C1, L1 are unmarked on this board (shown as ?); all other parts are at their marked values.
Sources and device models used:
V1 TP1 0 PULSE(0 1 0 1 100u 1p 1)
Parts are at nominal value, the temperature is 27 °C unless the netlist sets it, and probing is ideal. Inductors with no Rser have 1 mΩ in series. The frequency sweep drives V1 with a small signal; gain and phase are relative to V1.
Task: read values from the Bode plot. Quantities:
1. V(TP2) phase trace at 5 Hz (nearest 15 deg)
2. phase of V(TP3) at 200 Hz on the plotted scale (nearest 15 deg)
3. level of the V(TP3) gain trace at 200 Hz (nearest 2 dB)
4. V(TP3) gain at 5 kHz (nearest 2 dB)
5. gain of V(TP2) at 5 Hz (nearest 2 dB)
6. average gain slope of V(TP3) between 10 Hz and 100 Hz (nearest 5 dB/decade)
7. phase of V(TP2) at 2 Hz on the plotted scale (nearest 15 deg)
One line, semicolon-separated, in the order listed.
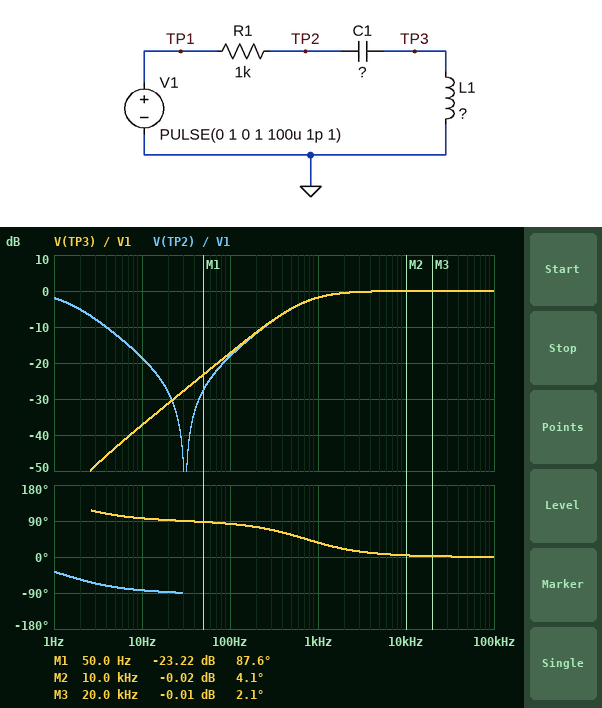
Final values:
-75 deg; 75 deg; -12 dB; 0 dB; -12 dB; 20 dB/decade; -60 deg
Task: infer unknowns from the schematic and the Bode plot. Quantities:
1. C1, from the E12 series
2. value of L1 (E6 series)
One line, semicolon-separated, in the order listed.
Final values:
120 µF; 220 mH
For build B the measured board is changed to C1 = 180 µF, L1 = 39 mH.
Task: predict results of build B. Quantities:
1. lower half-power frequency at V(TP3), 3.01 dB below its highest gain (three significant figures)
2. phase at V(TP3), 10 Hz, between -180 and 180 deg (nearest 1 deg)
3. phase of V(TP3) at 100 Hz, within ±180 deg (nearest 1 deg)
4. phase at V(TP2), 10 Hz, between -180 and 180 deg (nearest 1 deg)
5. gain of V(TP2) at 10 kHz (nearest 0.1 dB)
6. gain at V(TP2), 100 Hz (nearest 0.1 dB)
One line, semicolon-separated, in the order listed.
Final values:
4.08 kHz; 95 deg; 89 deg; -85 deg; -0.7 dB; -36.1 dB
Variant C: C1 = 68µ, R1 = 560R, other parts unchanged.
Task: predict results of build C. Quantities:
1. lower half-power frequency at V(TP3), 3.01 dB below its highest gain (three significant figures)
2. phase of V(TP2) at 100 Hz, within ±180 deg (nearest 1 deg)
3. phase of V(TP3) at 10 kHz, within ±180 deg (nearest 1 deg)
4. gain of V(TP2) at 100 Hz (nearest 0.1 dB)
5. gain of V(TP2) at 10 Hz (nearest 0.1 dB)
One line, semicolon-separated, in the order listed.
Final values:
401 Hz; 78 deg; 2 deg; -13.9 dB; -8.7 dB
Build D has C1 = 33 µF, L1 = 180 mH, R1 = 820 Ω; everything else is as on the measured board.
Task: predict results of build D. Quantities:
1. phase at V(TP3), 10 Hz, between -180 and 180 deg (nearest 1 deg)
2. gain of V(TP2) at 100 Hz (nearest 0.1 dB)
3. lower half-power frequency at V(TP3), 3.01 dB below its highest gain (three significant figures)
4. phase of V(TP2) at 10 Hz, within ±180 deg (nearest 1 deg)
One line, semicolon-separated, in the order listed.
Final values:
120 deg; -22.1 dB; 719 Hz; -60 deg
